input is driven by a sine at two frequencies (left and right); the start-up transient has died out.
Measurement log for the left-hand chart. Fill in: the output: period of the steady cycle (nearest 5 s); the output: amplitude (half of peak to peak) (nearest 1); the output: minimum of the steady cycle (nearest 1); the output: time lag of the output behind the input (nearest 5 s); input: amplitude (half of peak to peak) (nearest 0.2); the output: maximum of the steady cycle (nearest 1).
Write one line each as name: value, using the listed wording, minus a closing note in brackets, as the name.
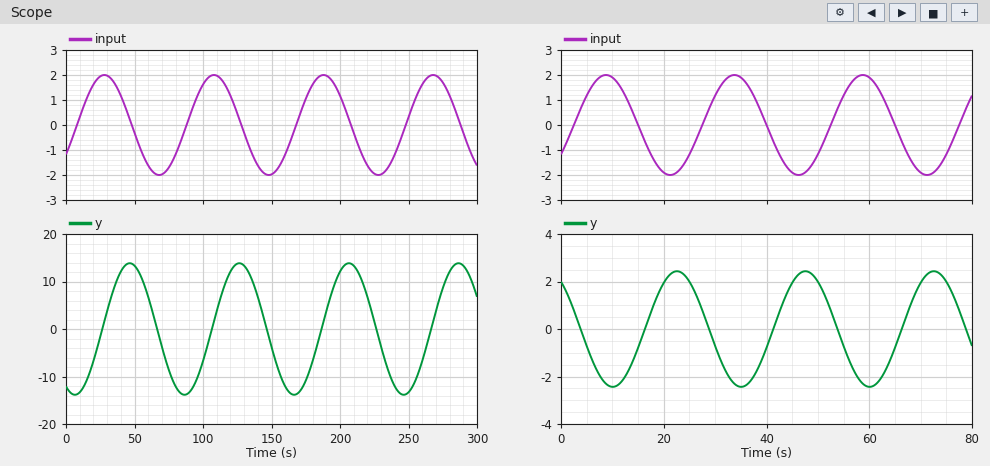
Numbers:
the output: period of the steady cycle: 80 s
the output: amplitude (half of peak to peak): 14
the output: minimum of the steady cycle: -14
the output: time lag of the output behind the input: 20 s
input: amplitude (half of peak to peak): 2.0
the output: maximum of the steady cycle: 14
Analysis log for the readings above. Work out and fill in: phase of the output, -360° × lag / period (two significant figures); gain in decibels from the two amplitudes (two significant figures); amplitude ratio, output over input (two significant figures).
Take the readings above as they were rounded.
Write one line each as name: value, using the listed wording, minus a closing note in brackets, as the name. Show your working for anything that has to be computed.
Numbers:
phase of the output, -360° × lag / period: -360 × 20 / 80 = -90°
gain in decibels from the two amplitudes: 20 log10(14 / 2) = 17 dB
amplitude ratio, output over input: 14 / 2 = 7.0
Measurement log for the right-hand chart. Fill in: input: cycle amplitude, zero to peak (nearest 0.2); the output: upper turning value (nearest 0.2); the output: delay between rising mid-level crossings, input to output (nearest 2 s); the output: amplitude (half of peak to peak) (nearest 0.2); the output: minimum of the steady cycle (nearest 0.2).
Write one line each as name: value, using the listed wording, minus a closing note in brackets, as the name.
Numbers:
input: cycle amplitude, zero to peak: 2.0
the output: upper turning value: 2.4
the output: delay between rising mid-level crossings, input to output: 14 s
the output: amplitude (half of peak to peak): 2.4
the output: minimum of the steady cycle: -2.4
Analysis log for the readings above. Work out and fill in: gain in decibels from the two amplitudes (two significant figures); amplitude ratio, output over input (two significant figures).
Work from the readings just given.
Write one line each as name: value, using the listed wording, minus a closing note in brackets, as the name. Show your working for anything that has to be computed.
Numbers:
gain in decibels from the two amplitudes: 20 log10(2.4 / 2) = 1.6 dB
amplitude ratio, output over input: 2.4 / 2 = 1.2
